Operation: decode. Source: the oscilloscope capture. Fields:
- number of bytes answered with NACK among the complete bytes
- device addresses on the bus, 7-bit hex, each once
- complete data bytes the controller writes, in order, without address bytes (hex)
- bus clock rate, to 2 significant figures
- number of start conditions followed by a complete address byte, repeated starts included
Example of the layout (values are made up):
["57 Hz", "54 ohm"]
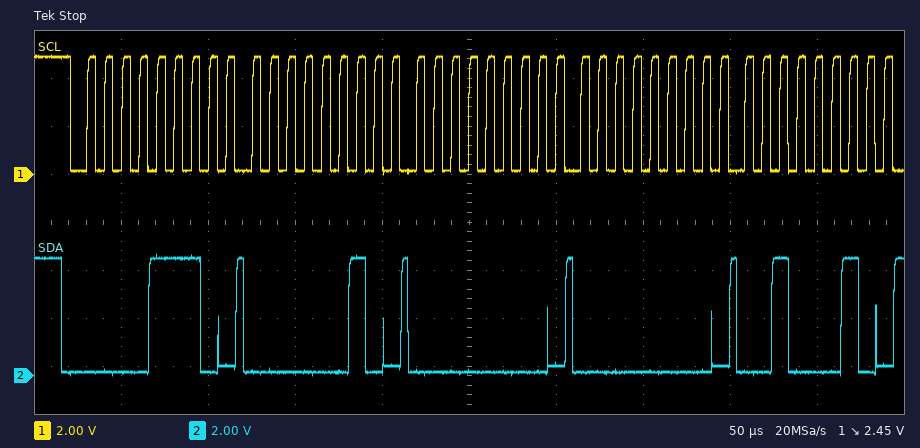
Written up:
["0", "0x07", "02 00 00 22", "100 kHz", "1"]
